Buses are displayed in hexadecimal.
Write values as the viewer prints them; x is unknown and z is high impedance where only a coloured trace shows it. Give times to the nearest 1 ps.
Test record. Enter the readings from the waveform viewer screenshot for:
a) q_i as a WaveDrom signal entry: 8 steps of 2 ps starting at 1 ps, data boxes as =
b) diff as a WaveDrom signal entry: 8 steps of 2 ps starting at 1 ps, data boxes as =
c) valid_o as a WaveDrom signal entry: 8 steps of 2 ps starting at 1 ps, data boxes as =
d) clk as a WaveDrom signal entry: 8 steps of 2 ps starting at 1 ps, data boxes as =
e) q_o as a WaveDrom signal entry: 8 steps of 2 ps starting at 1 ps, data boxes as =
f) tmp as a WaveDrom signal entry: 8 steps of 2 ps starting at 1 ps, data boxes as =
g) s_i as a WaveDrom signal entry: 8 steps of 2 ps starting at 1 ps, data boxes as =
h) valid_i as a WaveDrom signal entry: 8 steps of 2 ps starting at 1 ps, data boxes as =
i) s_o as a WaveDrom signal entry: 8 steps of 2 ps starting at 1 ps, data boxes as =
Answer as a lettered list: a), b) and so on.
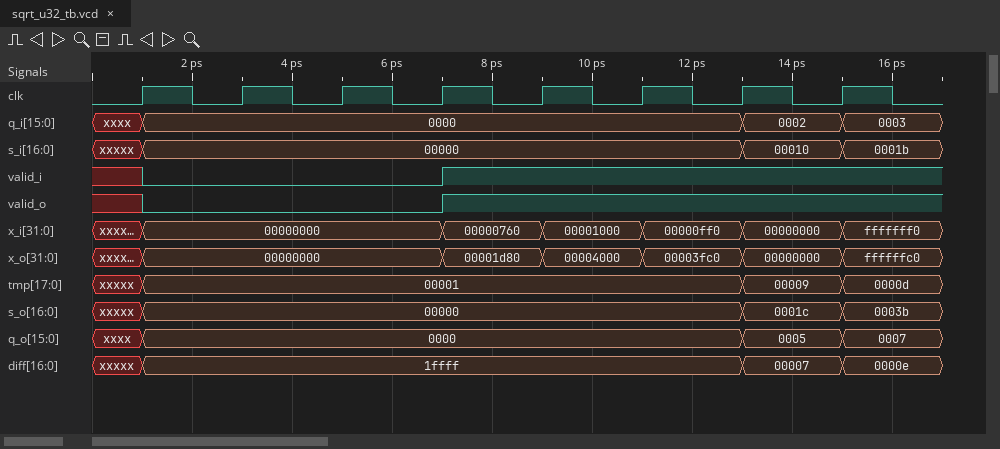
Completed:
a) {name: 'q_i', wave: '=.....==', data: '0000 0002 0003'}
b) {name: 'diff', wave: '=.....==', data: '1ffff 00007 0000e'}
c) {name: 'valid_o', wave: '0..1....'}
d) {name: 'clk', wave: 'p.......'}
e) {name: 'q_o', wave: '=.....==', data: '0000 0005 0007'}
f) {name: 'tmp', wave: '=.....==', data: '00001 00009 0000d'}
g) {name: 's_i', wave: '=.....==', data: '00000 00010 0001b'}
h) {name: 'valid_i', wave: '0..1....'}
i) {name: 's_o', wave: '=.....==', data: '00000 0001c 0003b'}
